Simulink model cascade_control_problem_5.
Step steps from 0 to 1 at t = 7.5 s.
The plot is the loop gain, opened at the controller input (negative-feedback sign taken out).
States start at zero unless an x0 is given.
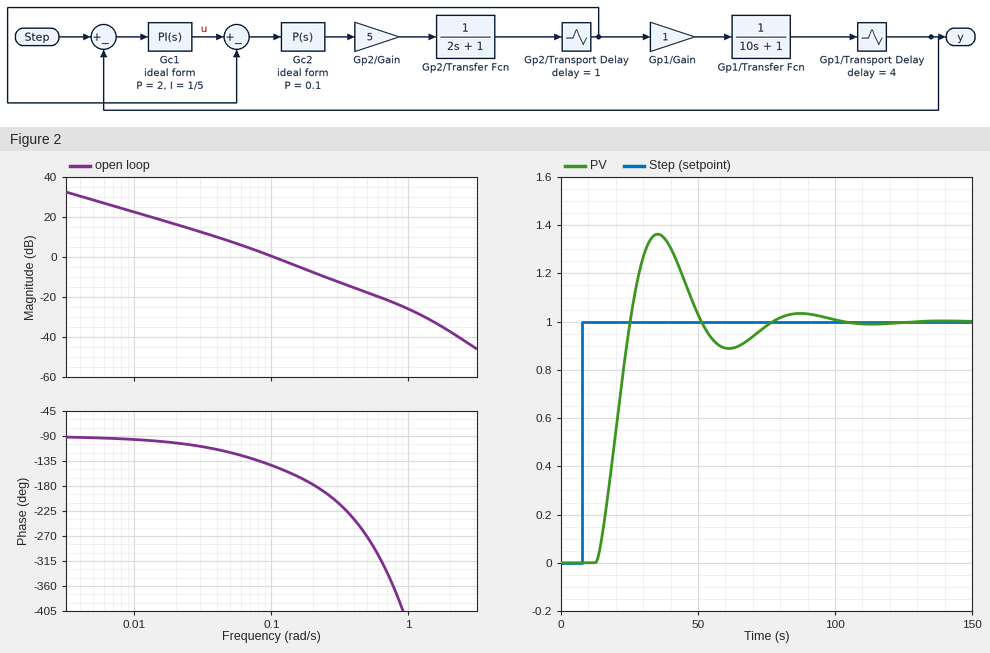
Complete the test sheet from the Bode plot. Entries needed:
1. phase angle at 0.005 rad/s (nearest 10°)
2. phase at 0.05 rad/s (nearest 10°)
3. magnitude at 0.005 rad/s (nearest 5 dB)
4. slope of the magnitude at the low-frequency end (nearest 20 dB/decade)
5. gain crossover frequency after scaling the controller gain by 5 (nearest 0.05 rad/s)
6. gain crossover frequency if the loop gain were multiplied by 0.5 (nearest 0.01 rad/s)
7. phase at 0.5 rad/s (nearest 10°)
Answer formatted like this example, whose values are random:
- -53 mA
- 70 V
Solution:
- -90°
- -120°
- 30 dB
- -20 dB/decade
- 0.35 rad/s
- 0.06 rad/s
- -270°
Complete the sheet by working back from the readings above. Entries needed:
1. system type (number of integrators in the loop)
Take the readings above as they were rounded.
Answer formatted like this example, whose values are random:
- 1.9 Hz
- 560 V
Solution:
- 1
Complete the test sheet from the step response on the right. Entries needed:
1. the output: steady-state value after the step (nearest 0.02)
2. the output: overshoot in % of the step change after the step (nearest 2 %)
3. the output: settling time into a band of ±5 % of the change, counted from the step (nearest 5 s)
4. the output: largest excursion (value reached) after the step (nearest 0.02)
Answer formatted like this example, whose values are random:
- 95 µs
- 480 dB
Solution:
- 1.00
- 36 %
- 65 s
- 1.36
